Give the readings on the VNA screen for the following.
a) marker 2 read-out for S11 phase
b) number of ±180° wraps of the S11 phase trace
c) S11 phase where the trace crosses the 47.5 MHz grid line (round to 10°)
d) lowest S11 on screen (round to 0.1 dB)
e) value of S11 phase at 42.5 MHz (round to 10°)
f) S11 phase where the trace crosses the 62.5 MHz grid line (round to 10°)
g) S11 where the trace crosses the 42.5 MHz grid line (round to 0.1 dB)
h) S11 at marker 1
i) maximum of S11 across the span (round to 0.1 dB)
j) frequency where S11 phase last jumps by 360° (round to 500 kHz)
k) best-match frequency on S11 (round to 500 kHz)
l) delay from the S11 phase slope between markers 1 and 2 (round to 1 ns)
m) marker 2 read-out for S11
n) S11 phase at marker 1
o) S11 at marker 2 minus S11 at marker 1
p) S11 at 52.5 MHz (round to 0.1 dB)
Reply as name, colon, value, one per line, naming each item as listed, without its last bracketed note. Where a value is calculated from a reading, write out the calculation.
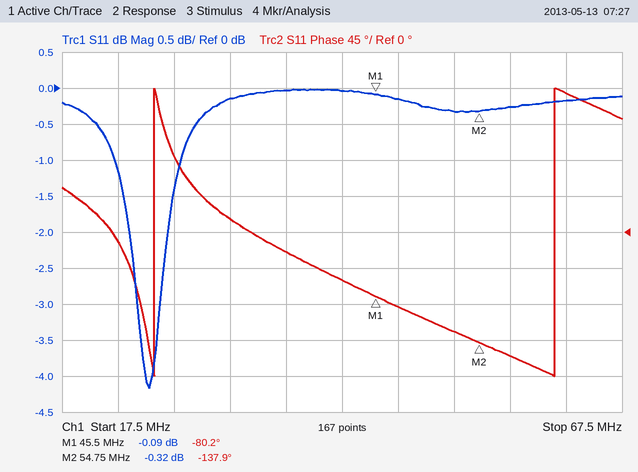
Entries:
marker 2 read-out for S11 phase: -137.9°
number of ±180° wraps of the S11 phase trace: 2
S11 phase where the trace crosses the 47.5 MHz grid line: -90°
lowest S11 on screen: -4.2 dB
value of S11 phase at 42.5 MHz: -60°
S11 phase where the trace crosses the 62.5 MHz grid line: 170°
S11 where the trace crosses the 42.5 MHz grid line: 0.0 dB
S11 at marker 1: -0.09 dB
maximum of S11 across the span: 0.0 dB
frequency where S11 phase last jumps by 360°: 61.5 MHz
best-match frequency on S11: 25.5 MHz
delay from the S11 phase slope between markers 1 and 2: −(-137.9° − (-80.2°))/(360° × 9.25 MHz) ≈ 17 ns
marker 2 read-out for S11: -0.32 dB
S11 phase at marker 1: -80.2°
S11 at marker 2 minus S11 at marker 1: -0.32 − (-0.09) = -0.23 dB
S11 at 52.5 MHz: -0.3 dB
